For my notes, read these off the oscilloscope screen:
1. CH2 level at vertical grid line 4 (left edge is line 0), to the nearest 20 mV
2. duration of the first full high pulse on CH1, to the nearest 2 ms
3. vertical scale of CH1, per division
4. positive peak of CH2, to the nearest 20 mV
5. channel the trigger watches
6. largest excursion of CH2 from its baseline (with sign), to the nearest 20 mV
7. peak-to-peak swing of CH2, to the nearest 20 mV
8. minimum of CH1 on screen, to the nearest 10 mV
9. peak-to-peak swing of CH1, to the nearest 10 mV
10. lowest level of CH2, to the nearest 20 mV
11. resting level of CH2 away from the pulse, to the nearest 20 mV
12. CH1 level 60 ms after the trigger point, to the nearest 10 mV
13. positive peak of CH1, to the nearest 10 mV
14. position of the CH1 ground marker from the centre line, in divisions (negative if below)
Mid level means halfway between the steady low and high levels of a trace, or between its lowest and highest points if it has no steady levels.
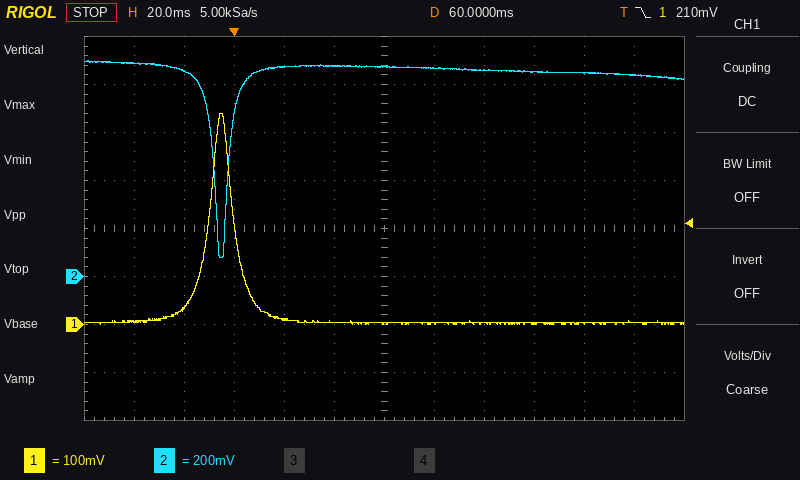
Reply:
880 mV
10 ms
100 mV
900 mV
CH1
-780 mV
820 mV
0 mV
440 mV
80 mV
860 mV
0 mV
440 mV
-2.0 div
